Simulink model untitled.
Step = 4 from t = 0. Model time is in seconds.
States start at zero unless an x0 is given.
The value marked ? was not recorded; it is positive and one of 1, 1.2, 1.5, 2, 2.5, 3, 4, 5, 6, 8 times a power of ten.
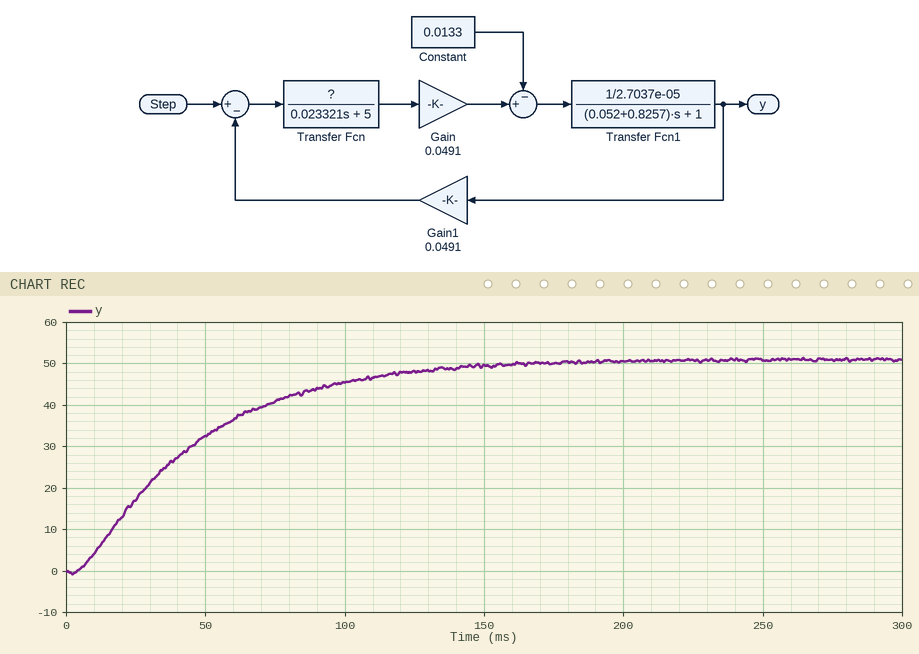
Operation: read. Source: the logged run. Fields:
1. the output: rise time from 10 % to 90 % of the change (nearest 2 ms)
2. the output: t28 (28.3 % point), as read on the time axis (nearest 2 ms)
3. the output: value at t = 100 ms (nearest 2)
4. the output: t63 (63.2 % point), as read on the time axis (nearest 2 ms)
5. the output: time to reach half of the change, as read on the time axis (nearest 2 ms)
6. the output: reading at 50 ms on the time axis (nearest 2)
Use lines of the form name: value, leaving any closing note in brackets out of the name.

the output: rise time from 10 % to 90 % of the change: 92 ms
the output: t28 (28.3 % point), as read on the time axis: 22 ms
the output: value at t = 100 ms: 46
the output: t63 (63.2 % point), as read on the time axis: 50 ms
the output: time to reach half of the change, as read on the time axis: 36 ms
the output: reading at 50 ms on the time axis: 32
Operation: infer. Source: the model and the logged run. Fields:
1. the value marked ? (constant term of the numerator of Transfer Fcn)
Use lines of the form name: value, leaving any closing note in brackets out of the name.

the value marked ?: 1
